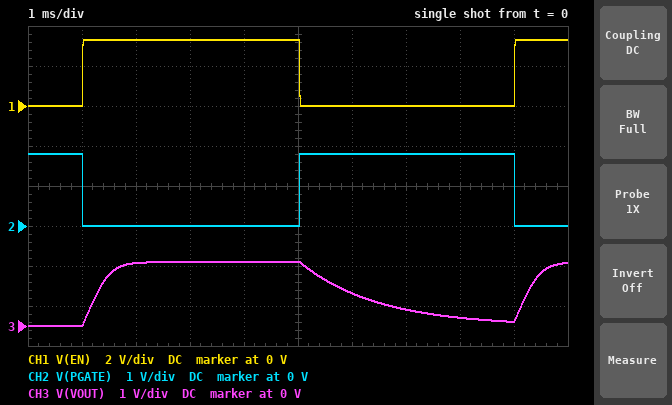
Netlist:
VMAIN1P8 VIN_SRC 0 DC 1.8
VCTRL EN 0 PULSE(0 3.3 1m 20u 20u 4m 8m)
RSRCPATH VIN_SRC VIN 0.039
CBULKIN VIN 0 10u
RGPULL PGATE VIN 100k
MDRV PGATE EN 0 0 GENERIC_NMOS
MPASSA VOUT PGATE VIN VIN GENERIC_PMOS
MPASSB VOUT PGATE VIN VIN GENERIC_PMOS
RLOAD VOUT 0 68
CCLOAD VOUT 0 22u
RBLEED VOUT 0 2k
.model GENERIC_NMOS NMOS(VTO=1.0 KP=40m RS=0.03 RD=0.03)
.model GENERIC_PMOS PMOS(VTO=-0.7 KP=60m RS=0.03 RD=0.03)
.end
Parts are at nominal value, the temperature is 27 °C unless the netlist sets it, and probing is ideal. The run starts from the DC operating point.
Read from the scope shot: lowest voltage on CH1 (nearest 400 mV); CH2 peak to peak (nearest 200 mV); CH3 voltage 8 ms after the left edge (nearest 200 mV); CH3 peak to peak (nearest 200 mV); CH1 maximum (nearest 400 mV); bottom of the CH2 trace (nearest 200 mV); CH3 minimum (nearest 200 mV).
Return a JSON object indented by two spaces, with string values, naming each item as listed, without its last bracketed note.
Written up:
{
  "lowest voltage on CH1": "0 V",
  "CH2 peak to peak": "1.8 V",
  "CH3 voltage 8 ms after the left edge": "200 mV",
  "CH3 peak to peak": "1.6 V",
  "CH1 maximum": "3.2 V",
  "bottom of the CH2 trace": "0 V",
  "CH3 minimum": "0 V"
}
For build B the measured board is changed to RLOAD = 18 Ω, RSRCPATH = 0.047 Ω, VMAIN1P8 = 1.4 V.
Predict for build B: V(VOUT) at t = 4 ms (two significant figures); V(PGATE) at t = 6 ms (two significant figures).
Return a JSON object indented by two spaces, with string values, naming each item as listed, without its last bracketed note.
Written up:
{
  "V(VOUT) at t = 4 ms": "520 mV",
  "V(PGATE) at t = 6 ms": "1.4 V"
}
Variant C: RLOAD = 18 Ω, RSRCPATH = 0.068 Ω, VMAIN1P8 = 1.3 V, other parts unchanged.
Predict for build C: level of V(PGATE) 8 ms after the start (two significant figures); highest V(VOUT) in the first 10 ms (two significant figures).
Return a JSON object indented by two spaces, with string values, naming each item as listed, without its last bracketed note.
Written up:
{
  "level of V(PGATE) 8 ms after the start": "1.3 V",
  "highest V(VOUT) in the first 10 ms": "380 mV"
}
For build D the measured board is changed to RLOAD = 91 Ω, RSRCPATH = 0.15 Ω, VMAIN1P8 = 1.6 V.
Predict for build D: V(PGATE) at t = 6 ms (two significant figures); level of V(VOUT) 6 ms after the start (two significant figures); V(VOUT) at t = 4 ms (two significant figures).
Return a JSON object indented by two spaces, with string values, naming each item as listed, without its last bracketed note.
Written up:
{
  "V(PGATE) at t = 6 ms": "1.6 V",
  "level of V(VOUT) 6 ms after the start": "860 mV",
  "V(VOUT) at t = 4 ms": "1.4 V"
}
